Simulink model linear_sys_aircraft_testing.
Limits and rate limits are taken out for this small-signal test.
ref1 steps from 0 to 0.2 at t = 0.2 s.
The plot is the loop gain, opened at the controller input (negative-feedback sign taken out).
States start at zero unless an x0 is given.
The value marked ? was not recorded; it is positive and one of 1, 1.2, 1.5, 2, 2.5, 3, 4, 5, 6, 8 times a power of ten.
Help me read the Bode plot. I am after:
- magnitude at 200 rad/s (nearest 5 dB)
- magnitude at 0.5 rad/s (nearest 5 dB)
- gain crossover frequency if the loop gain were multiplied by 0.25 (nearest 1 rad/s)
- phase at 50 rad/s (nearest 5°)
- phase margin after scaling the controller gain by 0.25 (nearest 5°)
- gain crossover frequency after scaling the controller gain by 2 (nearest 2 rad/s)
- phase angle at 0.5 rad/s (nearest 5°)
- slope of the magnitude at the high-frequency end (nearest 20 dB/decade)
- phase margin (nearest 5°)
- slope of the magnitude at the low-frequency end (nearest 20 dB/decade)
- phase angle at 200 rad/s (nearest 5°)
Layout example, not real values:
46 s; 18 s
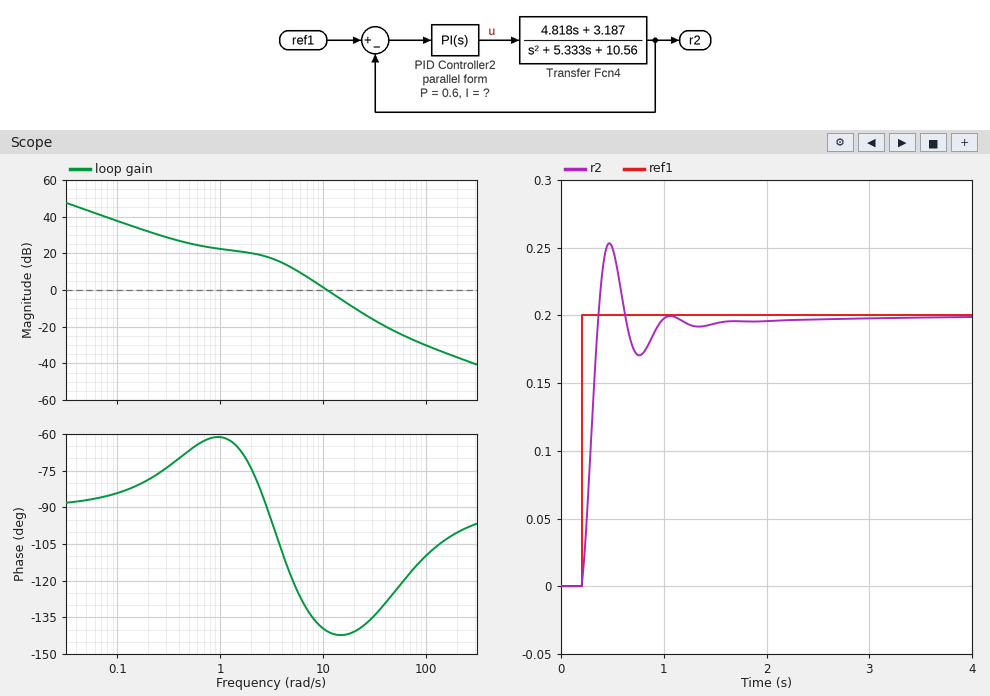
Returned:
-35 dB; 25 dB; 5 rad/s; -125°; 60°; 16 rad/s; -65°; -20 dB/decade; 40°; -20 dB/decade; -100°
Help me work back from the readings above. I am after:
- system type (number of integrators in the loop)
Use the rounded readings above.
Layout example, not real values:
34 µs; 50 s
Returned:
1
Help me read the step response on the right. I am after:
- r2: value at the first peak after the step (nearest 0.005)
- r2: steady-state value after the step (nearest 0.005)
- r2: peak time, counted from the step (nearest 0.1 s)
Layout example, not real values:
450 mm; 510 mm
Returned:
0.255; 0.200; 0.3 s
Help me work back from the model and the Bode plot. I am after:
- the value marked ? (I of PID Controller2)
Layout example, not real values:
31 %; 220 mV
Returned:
25
